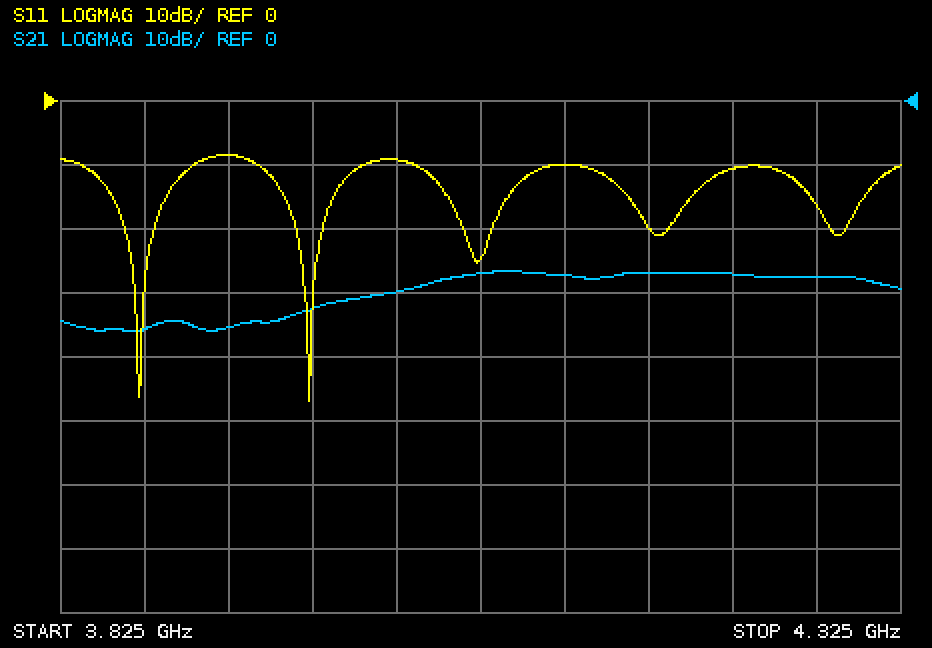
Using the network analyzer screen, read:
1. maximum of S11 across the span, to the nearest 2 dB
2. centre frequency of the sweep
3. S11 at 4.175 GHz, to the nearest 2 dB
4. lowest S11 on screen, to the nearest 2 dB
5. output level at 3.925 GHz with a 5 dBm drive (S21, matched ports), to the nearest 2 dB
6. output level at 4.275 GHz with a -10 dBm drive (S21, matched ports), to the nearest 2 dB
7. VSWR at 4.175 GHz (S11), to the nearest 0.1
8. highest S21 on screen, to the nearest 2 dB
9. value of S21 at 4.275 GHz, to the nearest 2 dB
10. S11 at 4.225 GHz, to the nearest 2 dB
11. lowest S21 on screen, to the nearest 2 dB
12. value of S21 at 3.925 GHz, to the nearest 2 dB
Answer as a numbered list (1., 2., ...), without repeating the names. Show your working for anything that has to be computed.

1. -8 dB
2. 4.075 GHz
3. -20 dB
4. -46 dB
5. 5 dBm + (-36 dB) = -30 dBm
6. -10 dBm + (-28 dB) = -38 dBm
7. |Γ| = 10^(-20/20) = 0.1000; VSWR = (1 + 0.1000)/(1 − 0.1000) ≈ 1.2
8. -26 dB
9. -28 dB
10. -10 dB
11. -36 dB
12. -36 dB
